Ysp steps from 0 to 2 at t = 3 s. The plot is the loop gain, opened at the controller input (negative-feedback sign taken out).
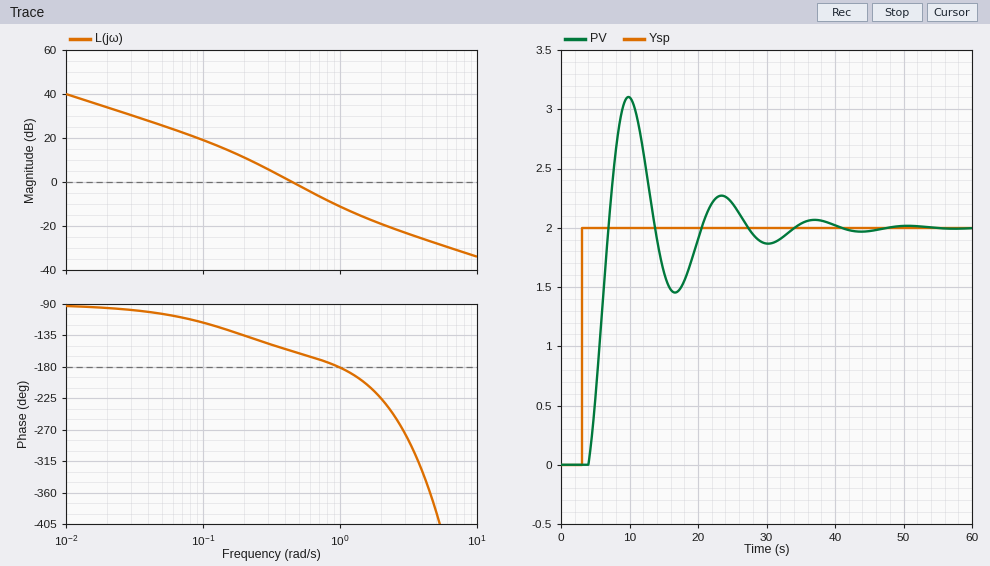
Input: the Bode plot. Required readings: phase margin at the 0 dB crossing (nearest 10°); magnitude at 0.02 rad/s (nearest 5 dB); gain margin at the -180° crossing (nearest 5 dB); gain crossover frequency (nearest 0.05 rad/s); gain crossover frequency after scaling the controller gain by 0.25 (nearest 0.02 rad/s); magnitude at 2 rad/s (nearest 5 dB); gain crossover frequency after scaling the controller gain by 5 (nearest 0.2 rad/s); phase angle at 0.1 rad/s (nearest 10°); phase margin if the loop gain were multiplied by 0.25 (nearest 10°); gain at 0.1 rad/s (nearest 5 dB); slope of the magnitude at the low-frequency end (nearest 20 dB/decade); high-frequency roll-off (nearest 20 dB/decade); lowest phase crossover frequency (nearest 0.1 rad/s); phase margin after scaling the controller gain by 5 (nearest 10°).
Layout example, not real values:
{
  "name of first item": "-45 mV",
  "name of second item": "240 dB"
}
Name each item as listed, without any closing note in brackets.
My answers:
{
  "phase margin at the 0 dB crossing": "20°",
  "magnitude at 0.02 rad/s": "35 dB",
  "gain margin at the -180° crossing": "10 dB",
  "gain crossover frequency": "0.45 rad/s",
  "gain crossover frequency after scaling the controller gain by 0.25": "0.18 rad/s",
  "magnitude at 2 rad/s": "-20 dB",
  "gain crossover frequency after scaling the controller gain by 5": "1.2 rad/s",
  "phase angle at 0.1 rad/s": "-120°",
  "phase margin if the loop gain were multiplied by 0.25": "50°",
  "gain at 0.1 rad/s": "20 dB",
  "slope of the magnitude at the low-frequency end": "-20 dB/decade",
  "high-frequency roll-off": "-20 dB/decade",
  "lowest phase crossover frequency": "1.0 rad/s",
  "phase margin after scaling the controller gain by 5": "-10°"
}
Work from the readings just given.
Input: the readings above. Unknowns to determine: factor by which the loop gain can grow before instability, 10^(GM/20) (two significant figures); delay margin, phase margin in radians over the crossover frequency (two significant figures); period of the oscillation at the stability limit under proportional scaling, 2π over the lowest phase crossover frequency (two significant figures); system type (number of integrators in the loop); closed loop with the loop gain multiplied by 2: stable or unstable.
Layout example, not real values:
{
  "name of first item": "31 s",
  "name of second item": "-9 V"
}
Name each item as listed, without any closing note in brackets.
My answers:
{
  "factor by which the loop gain can grow before instability, 10^(GM/20)": "3.2",
  "delay margin, phase margin in radians over the crossover frequency": "0.78 s",
  "period of the oscillation at the stability limit under proportional scaling, 2π over the lowest phase crossover frequency": "6.3 s",
  "system type": "1",
  "closed loop with the loop gain multiplied by 2: stable or unstable": "stable"
}
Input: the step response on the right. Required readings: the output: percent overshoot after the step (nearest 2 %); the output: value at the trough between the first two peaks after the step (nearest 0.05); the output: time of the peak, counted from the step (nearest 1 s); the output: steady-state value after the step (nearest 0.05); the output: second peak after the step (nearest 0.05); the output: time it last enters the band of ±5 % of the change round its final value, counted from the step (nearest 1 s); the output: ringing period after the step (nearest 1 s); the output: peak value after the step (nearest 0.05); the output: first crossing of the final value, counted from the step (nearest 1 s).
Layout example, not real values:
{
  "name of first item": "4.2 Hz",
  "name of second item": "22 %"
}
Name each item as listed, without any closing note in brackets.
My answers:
{
  "the output: percent overshoot after the step": "56 %",
  "the output: value at the trough between the first two peaks after the step": "1.45",
  "the output: time of the peak, counted from the step": "7 s",
  "the output: steady-state value after the step": "2.00",
  "the output: second peak after the step": "2.25",
  "the output: time it last enters the band of ±5 % of the change round its final value, counted from the step": "29 s",
  "the output: ringing period after the step": "14 s",
  "the output: peak value after the step": "3.10",
  "the output: first crossing of the final value, counted from the step": "4 s"
}
